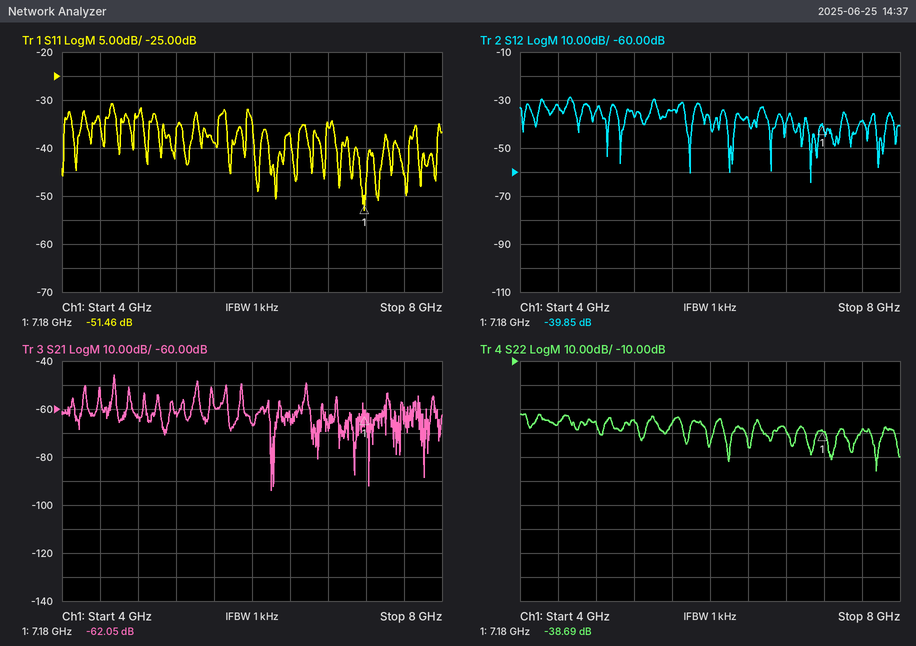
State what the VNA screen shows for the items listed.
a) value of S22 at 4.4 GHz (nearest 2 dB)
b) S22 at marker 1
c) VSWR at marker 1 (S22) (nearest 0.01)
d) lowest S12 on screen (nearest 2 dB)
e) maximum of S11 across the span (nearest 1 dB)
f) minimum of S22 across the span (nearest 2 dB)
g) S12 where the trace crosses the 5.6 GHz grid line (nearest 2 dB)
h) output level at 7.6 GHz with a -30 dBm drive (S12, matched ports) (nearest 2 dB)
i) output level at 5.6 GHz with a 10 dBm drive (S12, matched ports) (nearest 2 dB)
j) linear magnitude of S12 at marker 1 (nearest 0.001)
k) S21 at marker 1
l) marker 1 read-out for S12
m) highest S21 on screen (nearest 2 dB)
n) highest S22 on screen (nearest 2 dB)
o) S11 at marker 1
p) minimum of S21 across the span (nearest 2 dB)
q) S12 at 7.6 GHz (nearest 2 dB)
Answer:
-36 dB
-38.69 dB
1.02
-64 dB
-31 dB
-56 dB
-34 dB
-68 dBm
-24 dBm
0.010
-62.05 dB
-39.85 dB
-46 dB
-32 dB
-51.46 dB
-94 dB
-38 dB
